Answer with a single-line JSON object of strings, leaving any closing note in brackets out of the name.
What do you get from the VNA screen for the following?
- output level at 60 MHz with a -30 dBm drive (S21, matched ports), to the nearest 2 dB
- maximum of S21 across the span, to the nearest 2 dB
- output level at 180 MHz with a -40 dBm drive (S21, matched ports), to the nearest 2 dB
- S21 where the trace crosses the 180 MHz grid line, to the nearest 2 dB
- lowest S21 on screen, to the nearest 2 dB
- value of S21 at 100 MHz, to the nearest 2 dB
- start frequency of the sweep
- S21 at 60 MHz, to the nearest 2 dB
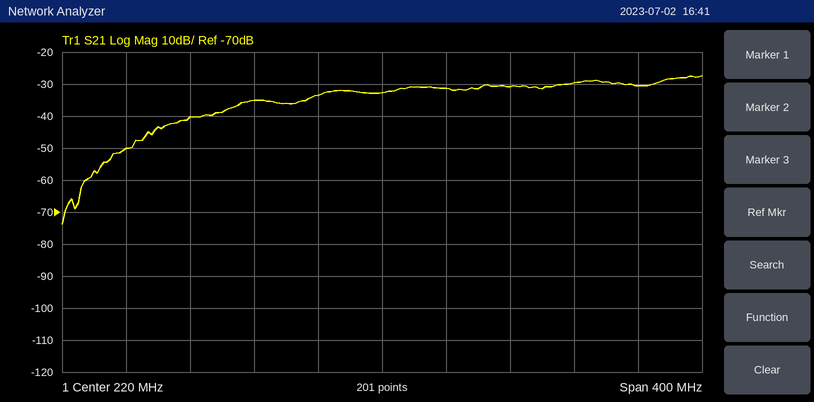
{"output level at 60 MHz with a -30 dBm drive (S21, matched ports), to the nearest 2 dB": "-80 dBm", "maximum of S21 across the span, to the nearest 2 dB": "-28 dB", "output level at 180 MHz with a -40 dBm drive (S21, matched ports), to the nearest 2 dB": "-74 dBm", "S21 where the trace crosses the 180 MHz grid line, to the nearest 2 dB": "-34 dB", "lowest S21 on screen, to the nearest 2 dB": "-74 dB", "value of S21 at 100 MHz, to the nearest 2 dB": "-40 dB", "start frequency of the sweep": "20 MHz", "S21 at 60 MHz, to the nearest 2 dB": "-50 dB"}
